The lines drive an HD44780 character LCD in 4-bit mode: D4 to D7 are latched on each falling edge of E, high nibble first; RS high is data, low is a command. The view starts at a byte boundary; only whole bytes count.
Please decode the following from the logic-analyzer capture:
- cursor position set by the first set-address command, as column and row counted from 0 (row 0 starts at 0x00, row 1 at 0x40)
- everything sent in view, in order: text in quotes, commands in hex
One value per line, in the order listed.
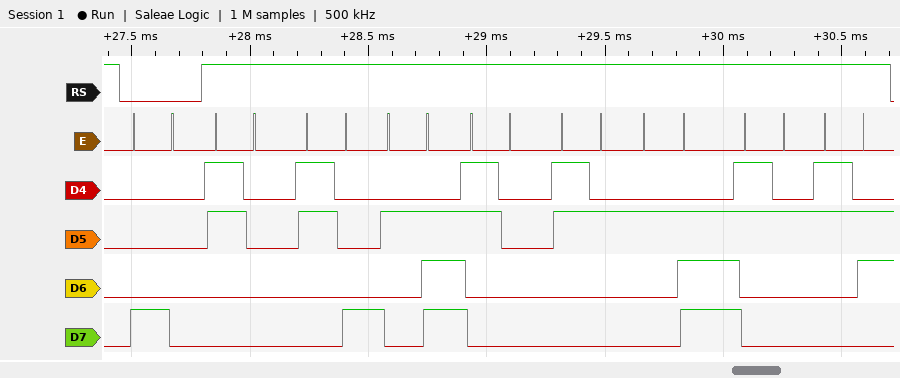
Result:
column 0, row 0
0x80 "08.02.26"
